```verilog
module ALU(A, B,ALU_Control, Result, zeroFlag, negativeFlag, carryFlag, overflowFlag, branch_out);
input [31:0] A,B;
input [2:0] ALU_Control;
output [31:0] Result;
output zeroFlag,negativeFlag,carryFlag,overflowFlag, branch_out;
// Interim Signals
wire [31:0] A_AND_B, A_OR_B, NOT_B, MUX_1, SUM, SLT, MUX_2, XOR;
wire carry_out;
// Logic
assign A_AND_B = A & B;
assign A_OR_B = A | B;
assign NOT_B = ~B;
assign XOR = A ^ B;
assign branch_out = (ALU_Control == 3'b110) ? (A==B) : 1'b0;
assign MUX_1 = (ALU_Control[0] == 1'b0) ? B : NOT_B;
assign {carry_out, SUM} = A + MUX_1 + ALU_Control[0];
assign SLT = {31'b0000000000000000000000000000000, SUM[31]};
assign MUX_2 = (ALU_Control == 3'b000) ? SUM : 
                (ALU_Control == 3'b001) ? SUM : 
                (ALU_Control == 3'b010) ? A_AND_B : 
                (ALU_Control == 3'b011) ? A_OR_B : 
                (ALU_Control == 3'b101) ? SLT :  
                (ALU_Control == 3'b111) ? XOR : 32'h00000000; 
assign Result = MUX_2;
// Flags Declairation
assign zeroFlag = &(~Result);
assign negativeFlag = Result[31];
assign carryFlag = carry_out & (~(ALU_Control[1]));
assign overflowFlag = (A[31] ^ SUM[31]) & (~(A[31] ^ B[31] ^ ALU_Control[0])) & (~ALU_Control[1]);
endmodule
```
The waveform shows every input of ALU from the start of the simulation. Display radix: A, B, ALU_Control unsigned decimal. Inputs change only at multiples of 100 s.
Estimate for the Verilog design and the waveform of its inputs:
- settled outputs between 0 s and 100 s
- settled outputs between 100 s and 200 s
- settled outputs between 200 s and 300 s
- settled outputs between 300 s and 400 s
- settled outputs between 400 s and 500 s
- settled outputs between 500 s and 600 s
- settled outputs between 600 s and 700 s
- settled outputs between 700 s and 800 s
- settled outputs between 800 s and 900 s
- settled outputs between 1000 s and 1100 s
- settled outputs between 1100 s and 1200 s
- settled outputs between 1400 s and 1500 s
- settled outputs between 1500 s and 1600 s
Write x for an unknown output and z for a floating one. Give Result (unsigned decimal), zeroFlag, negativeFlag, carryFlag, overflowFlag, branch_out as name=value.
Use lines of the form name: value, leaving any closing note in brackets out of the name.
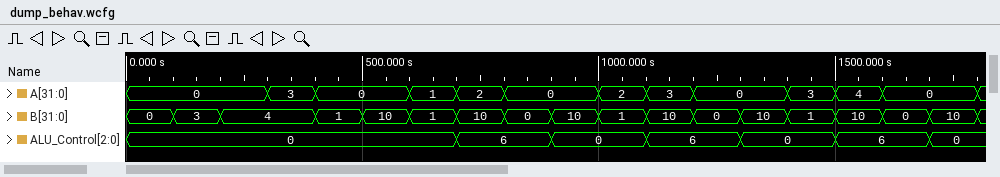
settled outputs between 0 s and 100 s: Result=0, zeroFlag=1, negativeFlag=0, carryFlag=0, overflowFlag=0, branch_out=0
settled outputs between 100 s and 200 s: Result=3, zeroFlag=0, negativeFlag=0, carryFlag=0, overflowFlag=0, branch_out=0
settled outputs between 200 s and 300 s: Result=4, zeroFlag=0, negativeFlag=0, carryFlag=0, overflowFlag=0, branch_out=0
settled outputs between 300 s and 400 s: Result=7, zeroFlag=0, negativeFlag=0, carryFlag=0, overflowFlag=0, branch_out=0
settled outputs between 400 s and 500 s: Result=1, zeroFlag=0, negativeFlag=0, carryFlag=0, overflowFlag=0, branch_out=0
settled outputs between 500 s and 600 s: Result=10, zeroFlag=0, negativeFlag=0, carryFlag=0, overflowFlag=0, branch_out=0
settled outputs between 600 s and 700 s: Result=2, zeroFlag=0, negativeFlag=0, carryFlag=0, overflowFlag=0, branch_out=0
settled outputs between 700 s and 800 s: Result=0, zeroFlag=1, negativeFlag=0, carryFlag=0, overflowFlag=0, branch_out=0
settled outputs between 800 s and 900 s: Result=0, zeroFlag=1, negativeFlag=0, carryFlag=0, overflowFlag=0, branch_out=1
settled outputs between 1000 s and 1100 s: Result=3, zeroFlag=0, negativeFlag=0, carryFlag=0, overflowFlag=0, branch_out=0
settled outputs between 1100 s and 1200 s: Result=0, zeroFlag=1, negativeFlag=0, carryFlag=0, overflowFlag=0, branch_out=0
settled outputs between 1400 s and 1500 s: Result=4, zeroFlag=0, negativeFlag=0, carryFlag=0, overflowFlag=0, branch_out=0
settled outputs between 1500 s and 1600 s: Result=0, zeroFlag=1, negativeFlag=0, carryFlag=0, overflowFlag=0, branch_out=0
